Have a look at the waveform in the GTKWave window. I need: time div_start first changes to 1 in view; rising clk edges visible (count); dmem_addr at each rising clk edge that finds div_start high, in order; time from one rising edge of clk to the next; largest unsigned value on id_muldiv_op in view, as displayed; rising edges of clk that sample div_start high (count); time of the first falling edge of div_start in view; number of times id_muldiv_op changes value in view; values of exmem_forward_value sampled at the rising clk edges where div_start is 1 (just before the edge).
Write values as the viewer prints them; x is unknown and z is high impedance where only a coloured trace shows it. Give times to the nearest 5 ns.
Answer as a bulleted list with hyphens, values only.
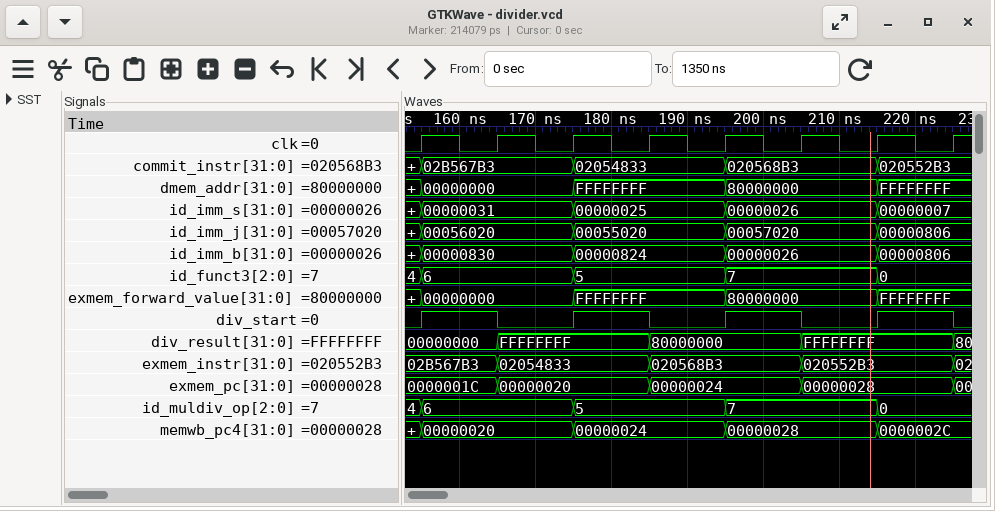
- 155 ns
- 8
- 00000000, FFFFFFFF, 80000000, FFFFFFFF
- 10 ns
- 7
- 4
- 165 ns
- 4
- 00000000, FFFFFFFF, 80000000, FFFFFFFF
